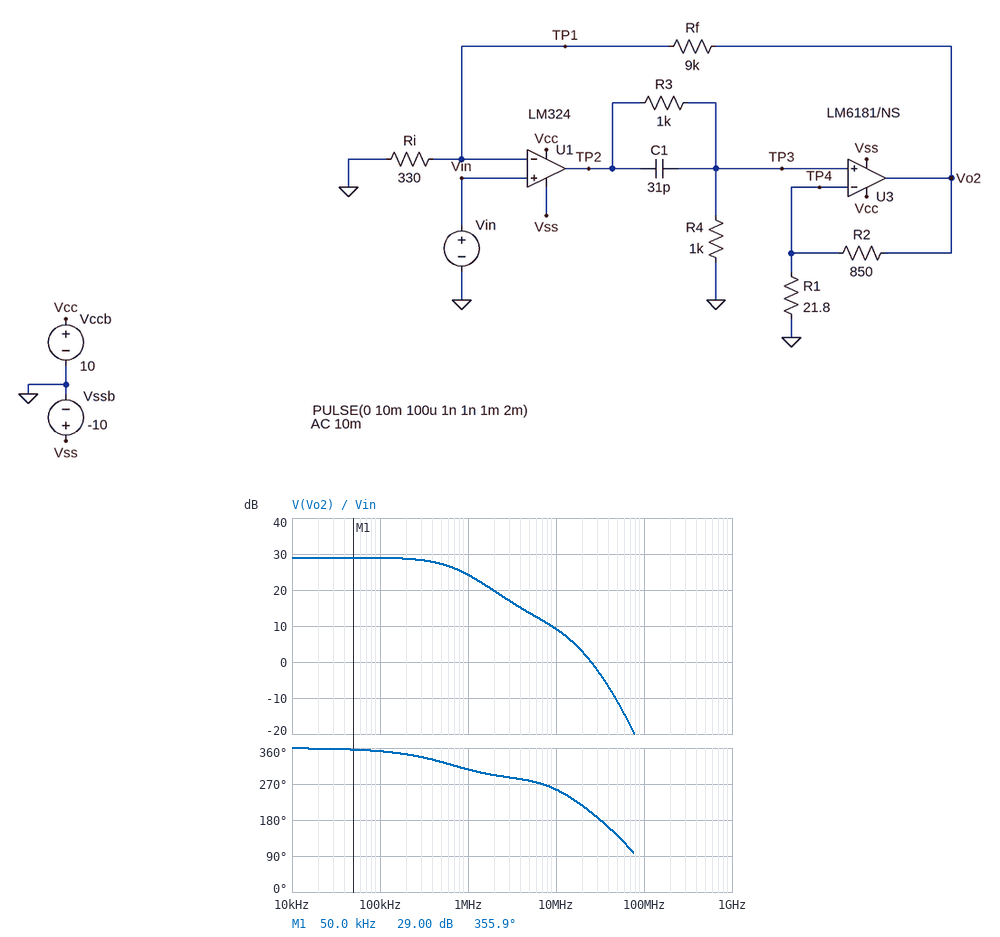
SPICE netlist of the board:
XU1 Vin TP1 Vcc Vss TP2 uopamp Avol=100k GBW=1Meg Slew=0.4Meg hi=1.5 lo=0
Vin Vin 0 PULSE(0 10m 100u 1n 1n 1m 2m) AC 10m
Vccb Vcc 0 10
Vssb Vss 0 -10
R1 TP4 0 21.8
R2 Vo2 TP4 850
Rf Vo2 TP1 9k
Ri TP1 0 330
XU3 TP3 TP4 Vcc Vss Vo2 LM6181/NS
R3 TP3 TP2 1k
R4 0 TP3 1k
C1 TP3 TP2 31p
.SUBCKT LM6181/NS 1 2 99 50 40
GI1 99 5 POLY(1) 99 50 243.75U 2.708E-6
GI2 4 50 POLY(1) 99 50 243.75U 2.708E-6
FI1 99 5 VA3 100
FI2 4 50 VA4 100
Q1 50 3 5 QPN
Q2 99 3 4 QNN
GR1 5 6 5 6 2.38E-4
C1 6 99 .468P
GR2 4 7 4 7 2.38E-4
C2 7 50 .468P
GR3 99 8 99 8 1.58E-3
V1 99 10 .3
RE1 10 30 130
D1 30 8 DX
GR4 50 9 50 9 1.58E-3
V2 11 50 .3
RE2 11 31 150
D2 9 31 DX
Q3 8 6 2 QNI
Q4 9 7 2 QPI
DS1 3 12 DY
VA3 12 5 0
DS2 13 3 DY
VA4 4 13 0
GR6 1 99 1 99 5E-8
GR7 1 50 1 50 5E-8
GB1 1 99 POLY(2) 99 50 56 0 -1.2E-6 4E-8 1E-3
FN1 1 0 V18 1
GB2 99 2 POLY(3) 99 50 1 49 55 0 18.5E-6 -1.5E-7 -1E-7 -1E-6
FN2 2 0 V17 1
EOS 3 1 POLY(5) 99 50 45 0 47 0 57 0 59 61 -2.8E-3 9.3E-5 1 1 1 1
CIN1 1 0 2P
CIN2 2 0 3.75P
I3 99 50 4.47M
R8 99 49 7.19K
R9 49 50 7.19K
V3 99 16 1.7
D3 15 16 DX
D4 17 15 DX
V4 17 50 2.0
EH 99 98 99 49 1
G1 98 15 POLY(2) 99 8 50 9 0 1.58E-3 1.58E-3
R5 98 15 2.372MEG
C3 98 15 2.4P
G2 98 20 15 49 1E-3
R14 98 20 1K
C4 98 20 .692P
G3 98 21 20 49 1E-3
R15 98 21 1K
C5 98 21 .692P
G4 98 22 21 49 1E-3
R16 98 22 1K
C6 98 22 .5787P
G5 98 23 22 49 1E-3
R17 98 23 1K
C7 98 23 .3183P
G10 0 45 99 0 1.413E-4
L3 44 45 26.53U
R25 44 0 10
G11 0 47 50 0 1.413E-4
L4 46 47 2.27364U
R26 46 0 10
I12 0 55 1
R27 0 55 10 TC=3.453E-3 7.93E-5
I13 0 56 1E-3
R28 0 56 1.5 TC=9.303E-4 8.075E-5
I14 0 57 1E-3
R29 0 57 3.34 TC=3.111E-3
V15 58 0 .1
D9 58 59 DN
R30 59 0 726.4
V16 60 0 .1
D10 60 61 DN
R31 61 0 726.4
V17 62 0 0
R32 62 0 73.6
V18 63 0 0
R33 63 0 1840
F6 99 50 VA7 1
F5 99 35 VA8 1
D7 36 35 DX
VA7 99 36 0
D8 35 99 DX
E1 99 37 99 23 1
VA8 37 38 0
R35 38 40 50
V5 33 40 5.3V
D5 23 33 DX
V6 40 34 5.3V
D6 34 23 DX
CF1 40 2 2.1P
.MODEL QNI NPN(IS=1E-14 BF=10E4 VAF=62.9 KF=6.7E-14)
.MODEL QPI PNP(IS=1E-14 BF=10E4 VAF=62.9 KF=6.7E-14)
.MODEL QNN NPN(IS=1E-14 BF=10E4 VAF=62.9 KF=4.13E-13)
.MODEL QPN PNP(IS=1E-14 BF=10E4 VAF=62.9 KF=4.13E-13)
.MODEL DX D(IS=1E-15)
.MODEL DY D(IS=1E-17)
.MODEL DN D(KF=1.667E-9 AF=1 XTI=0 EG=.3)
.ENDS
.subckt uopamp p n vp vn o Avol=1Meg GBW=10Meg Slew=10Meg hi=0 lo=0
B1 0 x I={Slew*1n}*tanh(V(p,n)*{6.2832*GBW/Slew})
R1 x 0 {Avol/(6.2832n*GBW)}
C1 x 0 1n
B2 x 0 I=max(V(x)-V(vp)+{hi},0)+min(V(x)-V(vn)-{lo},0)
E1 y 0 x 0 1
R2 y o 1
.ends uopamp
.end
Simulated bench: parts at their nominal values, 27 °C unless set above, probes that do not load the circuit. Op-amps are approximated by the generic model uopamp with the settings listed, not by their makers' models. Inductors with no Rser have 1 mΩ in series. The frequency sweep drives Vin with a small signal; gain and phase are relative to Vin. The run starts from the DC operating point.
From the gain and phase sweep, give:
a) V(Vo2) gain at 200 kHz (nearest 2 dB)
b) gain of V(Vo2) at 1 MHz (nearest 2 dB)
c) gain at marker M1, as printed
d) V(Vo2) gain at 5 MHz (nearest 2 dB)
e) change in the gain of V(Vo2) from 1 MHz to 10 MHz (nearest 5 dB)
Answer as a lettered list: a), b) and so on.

a) 28 dB
b) 24 dB
c) 29.00 dB
d) 14 dB
e) -15 dB
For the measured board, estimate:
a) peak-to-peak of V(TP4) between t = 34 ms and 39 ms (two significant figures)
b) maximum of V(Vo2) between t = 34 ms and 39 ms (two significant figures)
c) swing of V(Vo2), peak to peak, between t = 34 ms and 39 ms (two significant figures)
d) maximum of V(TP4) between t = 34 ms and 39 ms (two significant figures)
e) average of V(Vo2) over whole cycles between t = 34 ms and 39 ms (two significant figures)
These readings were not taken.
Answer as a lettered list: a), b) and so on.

a) 7.1 mV
b) 280 mV
c) 280 mV
d) 7.2 mV
e) 140 mV
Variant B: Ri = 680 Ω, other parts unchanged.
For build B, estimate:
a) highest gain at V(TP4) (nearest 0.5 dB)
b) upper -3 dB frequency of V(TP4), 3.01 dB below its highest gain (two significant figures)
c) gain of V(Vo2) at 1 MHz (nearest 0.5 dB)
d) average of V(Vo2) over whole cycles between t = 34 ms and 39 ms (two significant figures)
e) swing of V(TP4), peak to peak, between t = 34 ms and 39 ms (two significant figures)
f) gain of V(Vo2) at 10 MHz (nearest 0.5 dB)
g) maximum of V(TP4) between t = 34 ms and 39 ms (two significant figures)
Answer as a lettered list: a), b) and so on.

a) -9.0 dB
b) 1.4 MHz
c) 21.0 dB
d) 71 mV
e) 3.6 mV
f) 9.5 dB
g) 3.7 mV
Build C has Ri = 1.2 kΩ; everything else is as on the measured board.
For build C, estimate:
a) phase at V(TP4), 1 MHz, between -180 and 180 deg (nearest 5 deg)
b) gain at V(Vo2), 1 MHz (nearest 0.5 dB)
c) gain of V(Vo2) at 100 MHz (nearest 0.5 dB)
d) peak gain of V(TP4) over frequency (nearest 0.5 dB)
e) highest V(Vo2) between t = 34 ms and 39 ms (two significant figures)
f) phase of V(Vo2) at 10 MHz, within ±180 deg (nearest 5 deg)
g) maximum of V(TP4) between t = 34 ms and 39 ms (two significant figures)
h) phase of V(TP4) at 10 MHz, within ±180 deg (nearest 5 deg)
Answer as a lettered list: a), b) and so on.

a) -20 deg
b) 18.0 dB
c) -26.0 dB
d) -13.5 dB
e) 85 mV
f) -90 deg
g) 2.2 mV
h) -75 deg
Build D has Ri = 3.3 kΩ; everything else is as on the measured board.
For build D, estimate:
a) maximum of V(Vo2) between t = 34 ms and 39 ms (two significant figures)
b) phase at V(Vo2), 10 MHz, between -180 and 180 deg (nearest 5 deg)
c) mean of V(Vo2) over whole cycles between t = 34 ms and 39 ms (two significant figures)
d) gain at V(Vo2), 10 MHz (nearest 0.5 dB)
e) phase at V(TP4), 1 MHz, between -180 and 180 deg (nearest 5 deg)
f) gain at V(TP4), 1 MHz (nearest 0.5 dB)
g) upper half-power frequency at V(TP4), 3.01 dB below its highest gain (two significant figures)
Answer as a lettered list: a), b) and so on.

a) 37 mV
b) -65 deg
c) 19 mV
d) 8.5 dB
e) -10 deg
f) -21.0 dB
g) 12 MHz
